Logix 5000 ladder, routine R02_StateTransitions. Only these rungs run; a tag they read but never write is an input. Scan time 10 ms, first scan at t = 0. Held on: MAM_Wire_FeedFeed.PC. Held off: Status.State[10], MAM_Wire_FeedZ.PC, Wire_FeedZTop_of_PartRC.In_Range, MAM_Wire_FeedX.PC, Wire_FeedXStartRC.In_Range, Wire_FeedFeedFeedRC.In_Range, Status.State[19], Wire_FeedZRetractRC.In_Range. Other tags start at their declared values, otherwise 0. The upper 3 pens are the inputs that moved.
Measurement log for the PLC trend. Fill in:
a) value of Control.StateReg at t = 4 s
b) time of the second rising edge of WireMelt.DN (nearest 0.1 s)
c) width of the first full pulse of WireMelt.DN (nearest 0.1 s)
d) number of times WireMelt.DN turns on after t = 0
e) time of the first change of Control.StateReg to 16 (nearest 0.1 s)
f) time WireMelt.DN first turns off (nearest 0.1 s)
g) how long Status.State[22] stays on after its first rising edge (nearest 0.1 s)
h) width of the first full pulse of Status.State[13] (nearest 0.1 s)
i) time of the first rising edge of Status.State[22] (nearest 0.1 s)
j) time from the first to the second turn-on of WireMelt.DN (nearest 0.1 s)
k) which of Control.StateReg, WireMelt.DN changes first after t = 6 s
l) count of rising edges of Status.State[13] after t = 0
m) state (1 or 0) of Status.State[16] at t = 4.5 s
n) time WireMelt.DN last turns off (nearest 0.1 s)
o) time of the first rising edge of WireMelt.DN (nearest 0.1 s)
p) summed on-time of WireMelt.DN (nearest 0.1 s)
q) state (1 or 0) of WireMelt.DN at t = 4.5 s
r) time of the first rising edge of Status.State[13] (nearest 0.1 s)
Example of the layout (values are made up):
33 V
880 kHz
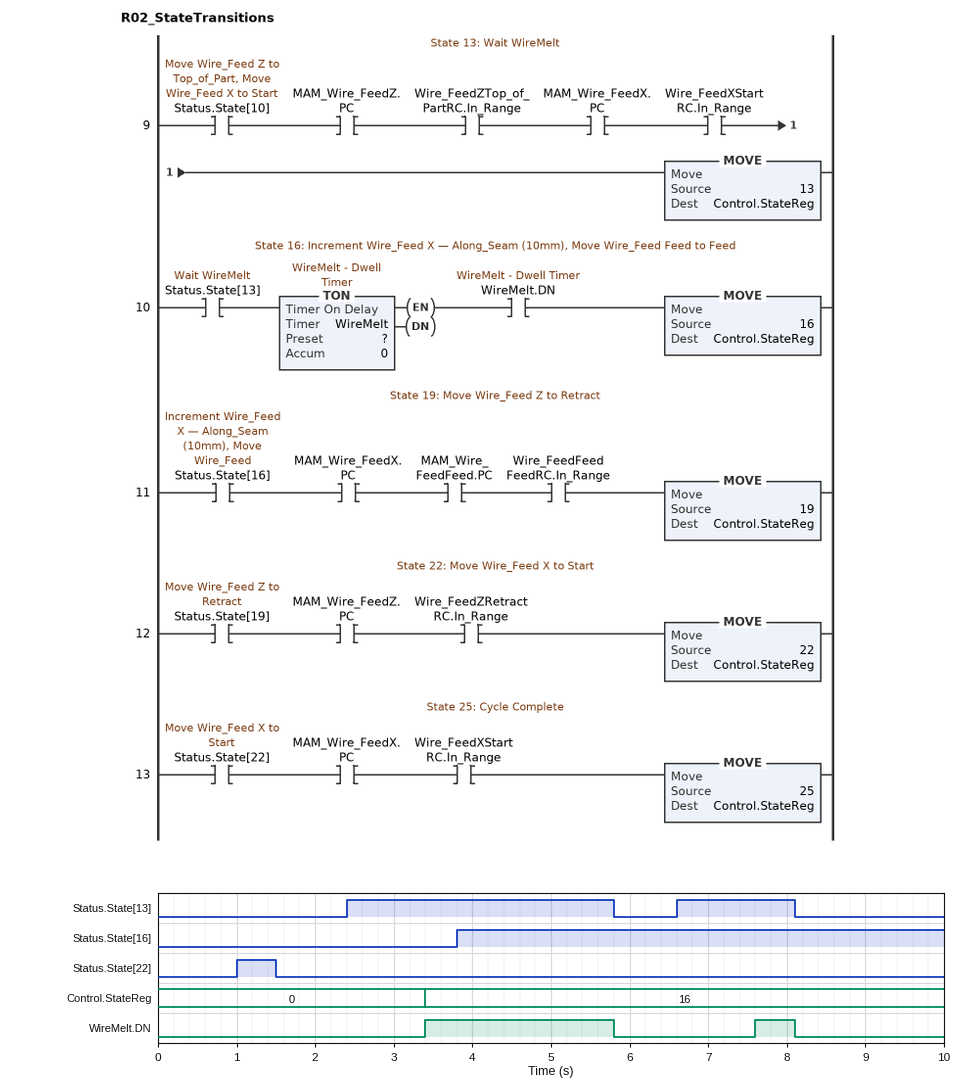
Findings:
16
7.6 s
2.4 s
2
3.4 s
5.8 s
0.5 s
3.4 s
1.0 s
4.2 s
WireMelt.DN
2
1
8.1 s
3.4 s
2.9 s
1
2.4 s
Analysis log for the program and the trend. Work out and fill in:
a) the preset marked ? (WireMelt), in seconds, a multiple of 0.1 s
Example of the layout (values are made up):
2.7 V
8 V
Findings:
1.0 s
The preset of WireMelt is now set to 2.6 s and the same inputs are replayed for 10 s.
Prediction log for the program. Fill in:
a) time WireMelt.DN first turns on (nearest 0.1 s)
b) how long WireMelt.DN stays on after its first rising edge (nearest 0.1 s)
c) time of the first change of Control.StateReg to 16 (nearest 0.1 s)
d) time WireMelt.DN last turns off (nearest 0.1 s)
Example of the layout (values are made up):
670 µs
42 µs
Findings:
5.0 s
0.8 s
5.0 s
5.8 s
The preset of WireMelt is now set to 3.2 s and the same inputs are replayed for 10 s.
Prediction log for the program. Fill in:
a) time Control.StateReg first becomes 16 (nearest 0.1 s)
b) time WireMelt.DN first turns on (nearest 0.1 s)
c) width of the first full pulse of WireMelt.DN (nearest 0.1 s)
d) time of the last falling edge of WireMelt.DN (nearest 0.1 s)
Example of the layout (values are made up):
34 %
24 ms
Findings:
5.6 s
5.6 s
0.2 s
5.8 s
